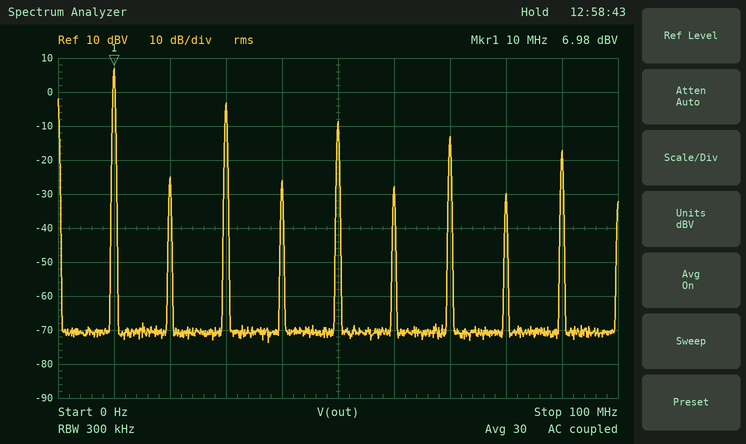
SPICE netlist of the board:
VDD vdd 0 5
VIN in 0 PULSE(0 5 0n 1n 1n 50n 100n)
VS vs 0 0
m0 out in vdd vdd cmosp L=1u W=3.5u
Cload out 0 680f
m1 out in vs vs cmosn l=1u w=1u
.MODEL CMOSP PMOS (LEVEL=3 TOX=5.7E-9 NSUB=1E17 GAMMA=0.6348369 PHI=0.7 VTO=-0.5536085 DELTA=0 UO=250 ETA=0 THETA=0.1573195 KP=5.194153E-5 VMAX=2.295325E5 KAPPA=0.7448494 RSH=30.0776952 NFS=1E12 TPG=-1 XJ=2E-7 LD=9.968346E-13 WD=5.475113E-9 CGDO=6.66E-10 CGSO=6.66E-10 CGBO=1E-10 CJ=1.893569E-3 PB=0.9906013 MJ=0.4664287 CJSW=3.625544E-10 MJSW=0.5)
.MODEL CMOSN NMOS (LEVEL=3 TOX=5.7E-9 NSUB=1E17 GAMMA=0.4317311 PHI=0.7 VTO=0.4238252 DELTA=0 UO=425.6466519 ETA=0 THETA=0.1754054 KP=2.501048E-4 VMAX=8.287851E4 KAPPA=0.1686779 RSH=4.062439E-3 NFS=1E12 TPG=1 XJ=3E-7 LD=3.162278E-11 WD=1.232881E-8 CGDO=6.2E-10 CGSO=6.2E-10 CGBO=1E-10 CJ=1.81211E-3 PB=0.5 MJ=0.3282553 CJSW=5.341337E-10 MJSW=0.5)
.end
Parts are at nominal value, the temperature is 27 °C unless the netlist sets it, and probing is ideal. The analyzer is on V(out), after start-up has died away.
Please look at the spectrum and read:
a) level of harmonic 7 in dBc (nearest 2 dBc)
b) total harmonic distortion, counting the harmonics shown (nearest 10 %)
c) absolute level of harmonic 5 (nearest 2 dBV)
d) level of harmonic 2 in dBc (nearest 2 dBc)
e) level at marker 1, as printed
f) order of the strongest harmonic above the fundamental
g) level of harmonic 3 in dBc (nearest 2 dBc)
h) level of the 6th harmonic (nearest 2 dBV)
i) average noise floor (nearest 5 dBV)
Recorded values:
-20 dBc
40 %
-8 dBV
-32 dBc
6.98 dBV
3
-10 dBc
-28 dBV
-70 dBV
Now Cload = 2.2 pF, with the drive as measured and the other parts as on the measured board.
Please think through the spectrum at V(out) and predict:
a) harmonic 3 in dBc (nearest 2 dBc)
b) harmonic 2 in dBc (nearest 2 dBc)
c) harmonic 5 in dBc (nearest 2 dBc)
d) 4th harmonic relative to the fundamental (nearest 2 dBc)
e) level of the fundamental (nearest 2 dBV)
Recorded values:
-14 dBc
-46 dBc
-26 dBc
-42 dBc
6 dBV
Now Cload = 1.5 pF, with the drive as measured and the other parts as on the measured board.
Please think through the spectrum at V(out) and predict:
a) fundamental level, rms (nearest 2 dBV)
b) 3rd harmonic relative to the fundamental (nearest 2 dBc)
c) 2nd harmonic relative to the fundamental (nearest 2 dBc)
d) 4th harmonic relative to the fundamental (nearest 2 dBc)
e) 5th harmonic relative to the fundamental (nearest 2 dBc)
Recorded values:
6 dBV
-12 dBc
-36 dBc
-42 dBc
-20 dBc
